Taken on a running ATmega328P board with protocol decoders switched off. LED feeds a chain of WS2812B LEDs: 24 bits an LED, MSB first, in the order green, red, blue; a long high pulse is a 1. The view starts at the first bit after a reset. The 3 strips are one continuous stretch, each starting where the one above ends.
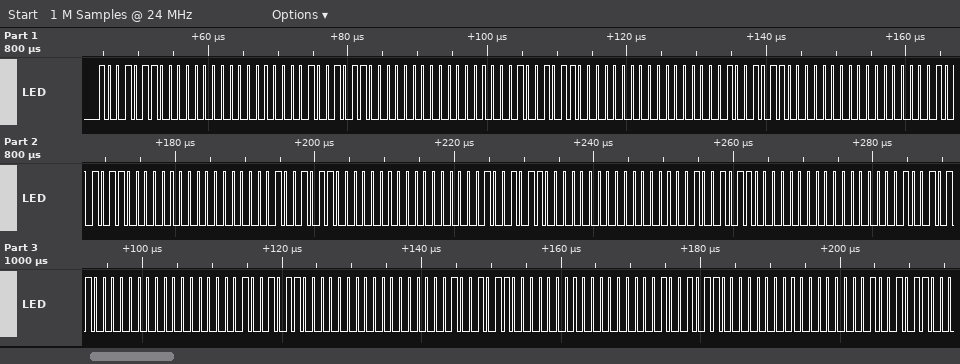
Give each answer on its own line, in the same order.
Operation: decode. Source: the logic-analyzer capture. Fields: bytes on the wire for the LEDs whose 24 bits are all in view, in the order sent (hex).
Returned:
96 00 00 96 00 00 96 00 00 96 00 00 96 00 00 96 00 00 96 00 00 96 00 00 96 00 00 96 00 00 96 00 00 96 00 00
